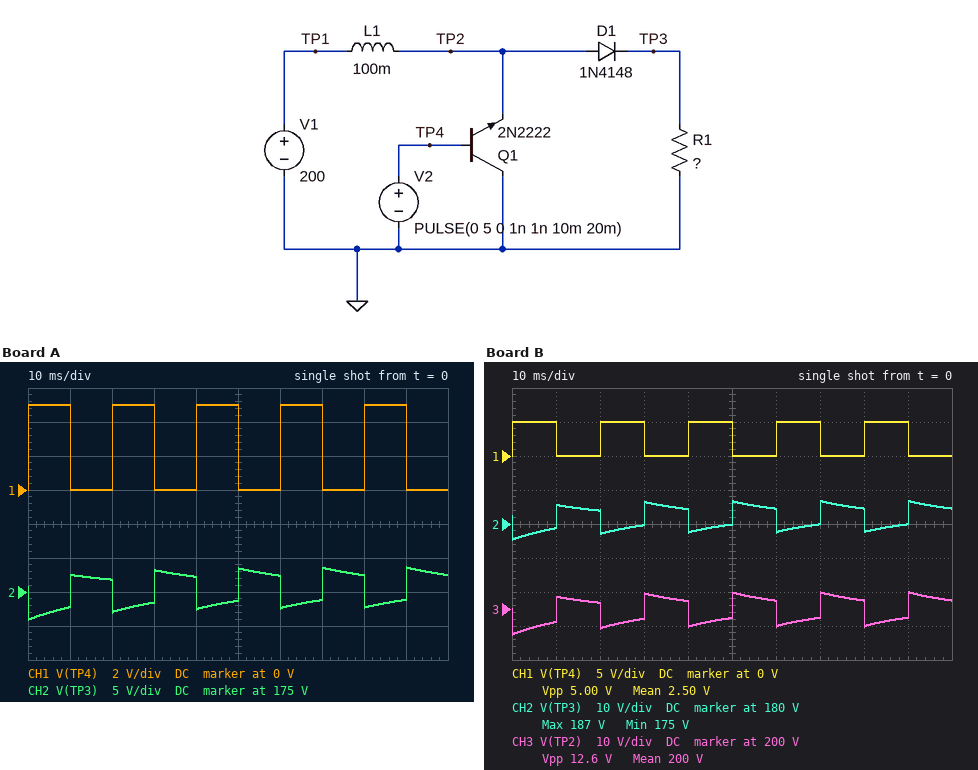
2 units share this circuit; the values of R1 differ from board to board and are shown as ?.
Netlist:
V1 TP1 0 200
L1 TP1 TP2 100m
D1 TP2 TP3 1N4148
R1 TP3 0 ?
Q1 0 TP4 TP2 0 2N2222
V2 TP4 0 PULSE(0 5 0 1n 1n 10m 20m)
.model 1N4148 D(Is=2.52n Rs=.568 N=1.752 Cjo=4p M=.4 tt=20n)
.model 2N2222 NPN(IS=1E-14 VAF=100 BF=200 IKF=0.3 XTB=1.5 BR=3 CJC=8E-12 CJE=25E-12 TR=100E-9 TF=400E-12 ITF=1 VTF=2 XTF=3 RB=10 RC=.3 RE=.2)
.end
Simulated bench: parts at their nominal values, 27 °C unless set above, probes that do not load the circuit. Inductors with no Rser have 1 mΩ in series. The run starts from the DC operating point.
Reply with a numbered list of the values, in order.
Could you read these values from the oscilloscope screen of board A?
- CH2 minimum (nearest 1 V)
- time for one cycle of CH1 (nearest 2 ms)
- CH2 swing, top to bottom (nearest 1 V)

1. 171 V
2. 20 ms
3. 8 V
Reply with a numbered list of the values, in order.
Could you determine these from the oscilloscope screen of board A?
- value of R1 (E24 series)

1. 4.3 Ω
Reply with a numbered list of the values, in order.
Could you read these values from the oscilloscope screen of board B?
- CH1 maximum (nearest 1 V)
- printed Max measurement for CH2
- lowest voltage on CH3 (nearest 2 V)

1. 5 V
2. 187 V
3. 192 V
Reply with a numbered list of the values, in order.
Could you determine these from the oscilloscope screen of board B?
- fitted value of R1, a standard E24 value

1. 6.2 Ω
